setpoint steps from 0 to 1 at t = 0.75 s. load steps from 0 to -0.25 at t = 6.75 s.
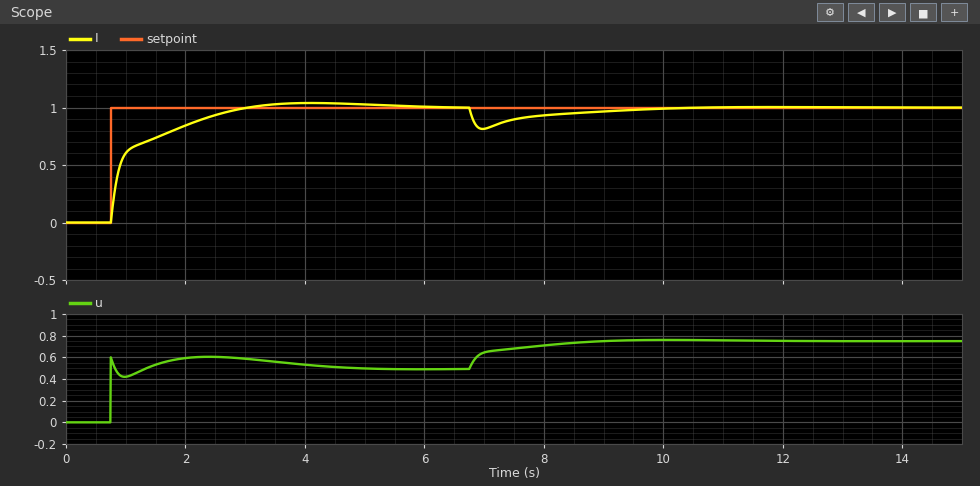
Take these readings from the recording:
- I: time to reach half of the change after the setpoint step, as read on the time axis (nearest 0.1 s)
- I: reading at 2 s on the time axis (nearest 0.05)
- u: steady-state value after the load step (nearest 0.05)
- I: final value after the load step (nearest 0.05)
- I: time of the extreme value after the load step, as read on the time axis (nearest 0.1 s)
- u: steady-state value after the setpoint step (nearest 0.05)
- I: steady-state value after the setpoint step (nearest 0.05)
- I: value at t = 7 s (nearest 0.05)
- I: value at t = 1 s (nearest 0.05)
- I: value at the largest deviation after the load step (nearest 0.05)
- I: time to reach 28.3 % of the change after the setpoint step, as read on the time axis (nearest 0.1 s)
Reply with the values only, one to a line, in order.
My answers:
0.9 s
0.85
0.75
1.00
7.0 s
0.50
1.00
0.80
0.60
0.80
0.8 s
